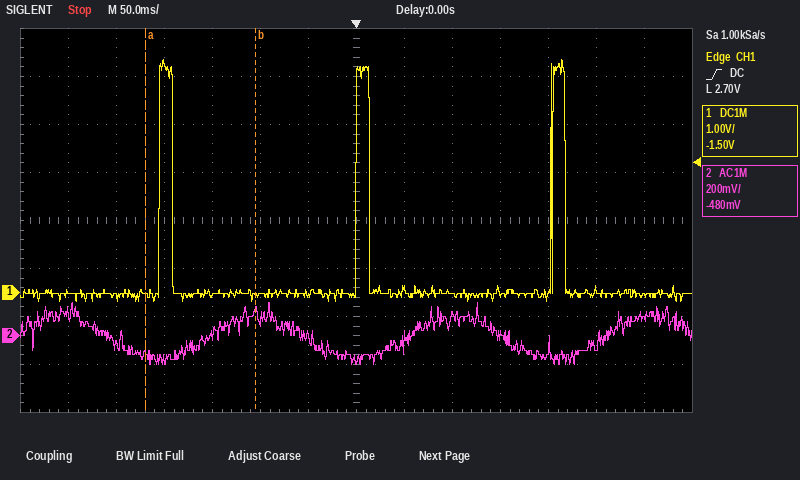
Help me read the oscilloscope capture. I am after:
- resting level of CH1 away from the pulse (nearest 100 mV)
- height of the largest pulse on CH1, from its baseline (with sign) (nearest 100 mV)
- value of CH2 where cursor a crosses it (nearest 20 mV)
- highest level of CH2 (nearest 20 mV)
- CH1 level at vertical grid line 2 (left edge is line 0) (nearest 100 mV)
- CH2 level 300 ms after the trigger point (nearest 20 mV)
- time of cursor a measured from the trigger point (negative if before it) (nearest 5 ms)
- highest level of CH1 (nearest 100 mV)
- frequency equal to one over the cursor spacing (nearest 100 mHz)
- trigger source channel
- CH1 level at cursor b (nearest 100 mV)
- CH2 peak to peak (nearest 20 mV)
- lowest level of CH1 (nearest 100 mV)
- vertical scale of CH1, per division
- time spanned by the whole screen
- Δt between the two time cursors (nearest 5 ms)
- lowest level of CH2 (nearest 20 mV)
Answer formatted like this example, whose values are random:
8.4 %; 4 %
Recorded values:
0.0 V; +4.9 V; -80 mV; 140 mV; -100 mV; 80 mV; -220 ms; 4.9 V; 8.7 Hz; CH1; -100 mV; 260 mV; -200 mV; 1 V; 700 ms; 115 ms; -120 mV
